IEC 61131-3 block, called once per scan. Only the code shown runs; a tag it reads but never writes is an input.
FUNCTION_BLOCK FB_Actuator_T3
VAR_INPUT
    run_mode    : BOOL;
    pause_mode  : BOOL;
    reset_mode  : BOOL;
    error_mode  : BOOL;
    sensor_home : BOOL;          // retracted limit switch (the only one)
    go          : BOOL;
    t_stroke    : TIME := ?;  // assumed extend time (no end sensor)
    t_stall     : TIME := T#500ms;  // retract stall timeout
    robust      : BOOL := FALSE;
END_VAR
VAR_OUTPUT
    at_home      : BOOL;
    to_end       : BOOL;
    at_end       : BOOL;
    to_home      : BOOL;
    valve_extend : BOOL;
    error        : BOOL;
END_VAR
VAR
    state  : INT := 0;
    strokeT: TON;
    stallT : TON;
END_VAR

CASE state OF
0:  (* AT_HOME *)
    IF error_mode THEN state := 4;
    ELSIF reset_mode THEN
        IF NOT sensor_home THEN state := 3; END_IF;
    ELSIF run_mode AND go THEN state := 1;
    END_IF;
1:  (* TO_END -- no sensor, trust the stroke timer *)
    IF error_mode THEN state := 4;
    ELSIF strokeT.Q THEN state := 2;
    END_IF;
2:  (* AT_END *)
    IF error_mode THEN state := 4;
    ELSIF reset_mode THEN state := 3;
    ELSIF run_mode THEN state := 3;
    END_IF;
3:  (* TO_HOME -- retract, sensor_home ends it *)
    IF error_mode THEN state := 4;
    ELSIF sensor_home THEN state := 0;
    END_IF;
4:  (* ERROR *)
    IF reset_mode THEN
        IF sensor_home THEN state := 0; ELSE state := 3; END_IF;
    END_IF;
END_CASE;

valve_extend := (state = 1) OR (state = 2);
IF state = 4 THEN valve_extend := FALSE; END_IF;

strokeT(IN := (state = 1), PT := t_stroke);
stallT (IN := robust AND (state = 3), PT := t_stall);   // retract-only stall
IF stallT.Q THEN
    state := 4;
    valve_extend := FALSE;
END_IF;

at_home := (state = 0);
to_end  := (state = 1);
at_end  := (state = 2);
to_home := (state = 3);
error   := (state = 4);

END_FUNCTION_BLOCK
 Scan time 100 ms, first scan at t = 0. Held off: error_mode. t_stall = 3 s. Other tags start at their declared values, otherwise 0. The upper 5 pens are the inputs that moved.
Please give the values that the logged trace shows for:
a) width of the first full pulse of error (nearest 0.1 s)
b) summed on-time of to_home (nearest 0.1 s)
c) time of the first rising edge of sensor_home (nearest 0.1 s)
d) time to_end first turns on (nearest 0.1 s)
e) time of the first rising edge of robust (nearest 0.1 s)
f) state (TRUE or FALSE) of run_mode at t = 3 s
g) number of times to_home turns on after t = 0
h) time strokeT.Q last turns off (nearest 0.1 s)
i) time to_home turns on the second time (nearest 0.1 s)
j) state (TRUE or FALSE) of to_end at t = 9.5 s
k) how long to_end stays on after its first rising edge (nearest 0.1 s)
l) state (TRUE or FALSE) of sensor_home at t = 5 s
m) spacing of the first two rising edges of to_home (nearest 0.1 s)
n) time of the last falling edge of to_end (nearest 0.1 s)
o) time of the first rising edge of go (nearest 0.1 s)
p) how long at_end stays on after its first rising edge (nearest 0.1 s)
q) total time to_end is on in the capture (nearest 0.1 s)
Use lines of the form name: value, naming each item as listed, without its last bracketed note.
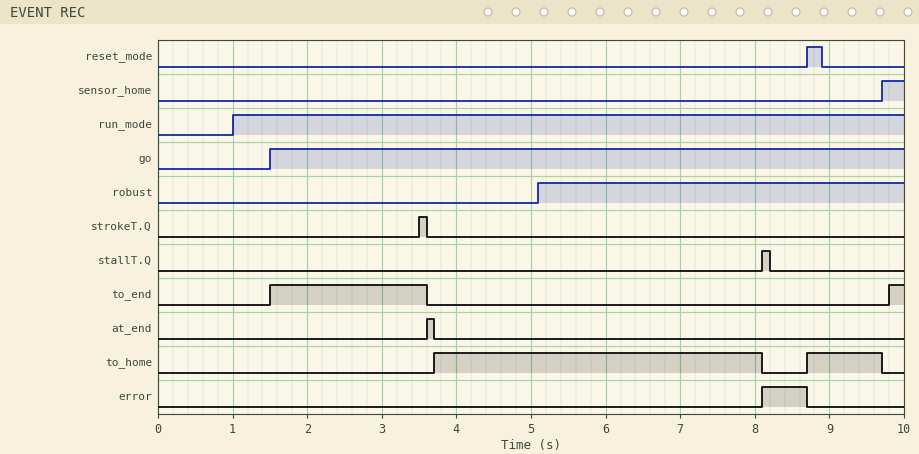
width of the first full pulse of error: 0.6 s
summed on-time of to_home: 5.4 s
time of the first rising edge of sensor_home: 9.7 s
time to_end first turns on: 1.5 s
time of the first rising edge of robust: 5.1 s
state (TRUE or FALSE) of run_mode at t = 3 s: TRUE
number of times to_home turns on after t = 0: 2
time strokeT.Q last turns off: 3.6 s
time to_home turns on the second time: 8.7 s
state (TRUE or FALSE) of to_end at t = 9.5 s: FALSE
how long to_end stays on after its first rising edge: 2.1 s
state (TRUE or FALSE) of sensor_home at t = 5 s: FALSE
spacing of the first two rising edges of to_home: 5.0 s
time of the last falling edge of to_end: 3.6 s
time of the first rising edge of go: 1.5 s
how long at_end stays on after its first rising edge: 0.1 s
total time to_end is on in the capture: 2.3 s
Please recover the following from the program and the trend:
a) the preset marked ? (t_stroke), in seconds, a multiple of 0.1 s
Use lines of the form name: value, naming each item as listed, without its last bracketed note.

the preset marked ? (t_stroke), in seconds, a multiple of 0.1 s: 2.0 s
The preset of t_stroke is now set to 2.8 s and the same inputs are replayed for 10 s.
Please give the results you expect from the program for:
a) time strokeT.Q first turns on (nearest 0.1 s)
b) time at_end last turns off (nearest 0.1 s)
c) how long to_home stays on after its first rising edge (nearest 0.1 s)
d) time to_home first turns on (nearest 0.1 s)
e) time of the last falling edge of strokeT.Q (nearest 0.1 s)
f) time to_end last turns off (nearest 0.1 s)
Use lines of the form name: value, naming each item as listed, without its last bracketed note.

time strokeT.Q first turns on: 4.3 s
time at_end last turns off: 4.5 s
how long to_home stays on after its first rising edge: 3.6 s
time to_home first turns on: 4.5 s
time of the last falling edge of strokeT.Q: 4.4 s
time to_end last turns off: 4.4 s
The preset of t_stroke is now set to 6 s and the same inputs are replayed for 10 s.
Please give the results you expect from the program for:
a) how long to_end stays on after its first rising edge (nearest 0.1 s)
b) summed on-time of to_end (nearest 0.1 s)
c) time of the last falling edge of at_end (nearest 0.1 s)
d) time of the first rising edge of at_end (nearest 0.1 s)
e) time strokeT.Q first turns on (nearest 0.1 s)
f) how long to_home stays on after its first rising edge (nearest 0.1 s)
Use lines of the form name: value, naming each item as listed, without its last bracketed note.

how long to_end stays on after its first rising edge: 6.1 s
summed on-time of to_end: 6.3 s
time of the last falling edge of at_end: 7.7 s
time of the first rising edge of at_end: 7.6 s
time strokeT.Q first turns on: 7.5 s
how long to_home stays on after its first rising edge: 2.0 s
